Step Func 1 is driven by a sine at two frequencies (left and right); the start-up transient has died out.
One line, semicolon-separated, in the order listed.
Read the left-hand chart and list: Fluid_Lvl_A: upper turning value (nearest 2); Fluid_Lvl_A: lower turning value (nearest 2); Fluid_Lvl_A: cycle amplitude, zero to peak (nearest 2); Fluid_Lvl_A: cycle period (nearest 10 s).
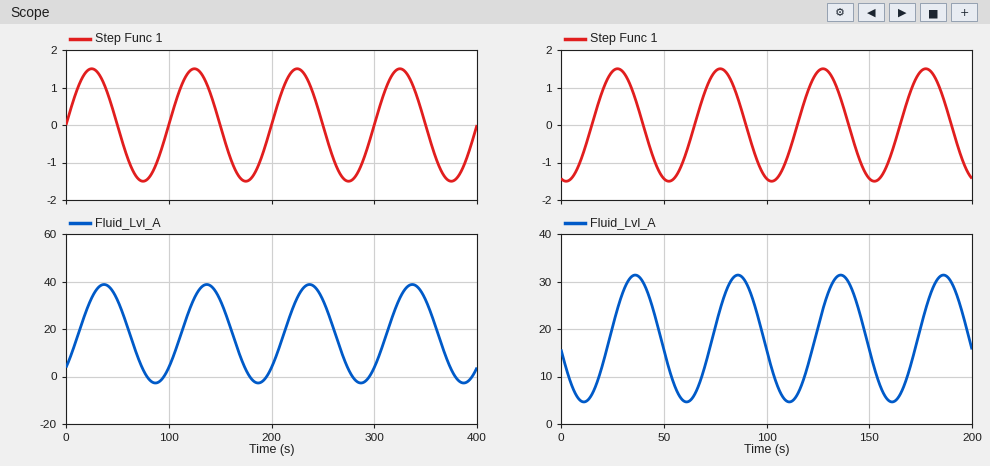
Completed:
38; -2; 20; 100 s
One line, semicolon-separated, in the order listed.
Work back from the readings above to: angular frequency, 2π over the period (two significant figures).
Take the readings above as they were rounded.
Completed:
0.063 rad/s
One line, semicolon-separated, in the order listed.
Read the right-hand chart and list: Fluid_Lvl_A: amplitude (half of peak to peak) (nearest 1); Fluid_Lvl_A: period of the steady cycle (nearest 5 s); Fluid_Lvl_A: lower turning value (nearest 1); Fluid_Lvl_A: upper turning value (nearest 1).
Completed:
13; 50 s; 5; 31
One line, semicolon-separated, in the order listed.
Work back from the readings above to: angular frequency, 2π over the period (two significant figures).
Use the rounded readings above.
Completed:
0.13 rad/s
